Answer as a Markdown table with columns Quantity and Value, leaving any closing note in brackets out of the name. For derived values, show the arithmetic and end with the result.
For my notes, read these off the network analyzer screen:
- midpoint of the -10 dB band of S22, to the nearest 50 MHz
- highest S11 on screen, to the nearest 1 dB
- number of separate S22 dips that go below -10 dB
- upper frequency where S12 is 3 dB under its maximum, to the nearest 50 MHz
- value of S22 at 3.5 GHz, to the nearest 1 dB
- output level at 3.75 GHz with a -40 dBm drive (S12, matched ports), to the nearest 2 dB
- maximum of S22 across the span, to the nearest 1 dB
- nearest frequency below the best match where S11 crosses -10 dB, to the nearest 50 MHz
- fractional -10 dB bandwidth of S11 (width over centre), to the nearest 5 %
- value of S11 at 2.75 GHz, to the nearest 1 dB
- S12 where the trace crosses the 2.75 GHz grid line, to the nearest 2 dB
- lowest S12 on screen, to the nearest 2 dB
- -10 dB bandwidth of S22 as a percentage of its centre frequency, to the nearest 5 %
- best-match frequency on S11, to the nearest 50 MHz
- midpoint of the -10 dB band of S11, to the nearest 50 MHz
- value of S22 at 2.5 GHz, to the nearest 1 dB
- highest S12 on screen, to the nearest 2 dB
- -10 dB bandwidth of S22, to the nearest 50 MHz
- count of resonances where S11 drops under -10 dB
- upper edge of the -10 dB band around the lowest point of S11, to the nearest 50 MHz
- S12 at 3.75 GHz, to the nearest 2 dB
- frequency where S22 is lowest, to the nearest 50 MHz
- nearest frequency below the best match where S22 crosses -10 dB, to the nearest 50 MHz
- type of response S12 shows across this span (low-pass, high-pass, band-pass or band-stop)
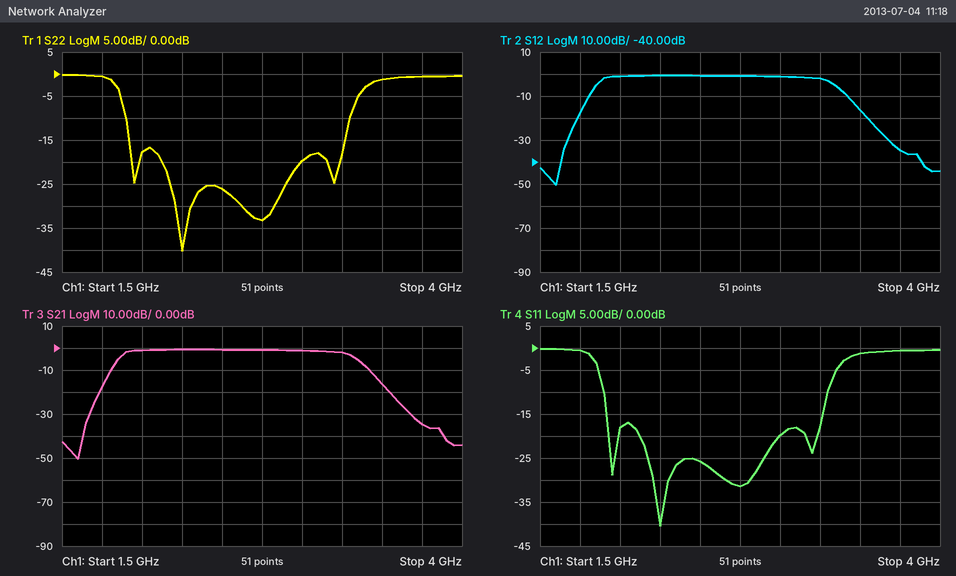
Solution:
| Quantity | Value |
|---|---|
| midpoint of the -10 dB band of S22, to the nearest 50 MHz | 2.60 GHz |
| highest S11 on screen, to the nearest 1 dB | 0 dB |
| number of separate S22 dips that go below -10 dB | 4 |
| upper frequency where S12 is 3 dB under its maximum, to the nearest 50 MHz | 3.30 GHz |
| value of S22 at 3.5 GHz, to the nearest 1 dB | -1 dB |
| output level at 3.75 GHz with a -40 dBm drive (S12, matched ports), to the nearest 2 dB | -40 dBm + (-34 dB) = -74 dBm |
| maximum of S22 across the span, to the nearest 1 dB | 0 dB |
| nearest frequency below the best match where S11 crosses -10 dB, to the nearest 50 MHz | 1.90 GHz |
| fractional -10 dB bandwidth of S11 (width over centre), to the nearest 5 % | 1.4 GHz / 2.6 GHz ≈ 53.8 %, so 55 % to the nearest 5 % |
| value of S11 at 2.75 GHz, to the nearest 1 dB | -31 dB |
| S12 where the trace crosses the 2.75 GHz grid line, to the nearest 2 dB | 0 dB |
| lowest S12 on screen, to the nearest 2 dB | -50 dB |
| -10 dB bandwidth of S22 as a percentage of its centre frequency, to the nearest 5 % | 1.4 GHz / 2.6 GHz ≈ 53.8 %, so 55 % to the nearest 5 % |
| best-match frequency on S11, to the nearest 50 MHz | 2.25 GHz |
| midpoint of the -10 dB band of S11, to the nearest 50 MHz | 2.60 GHz |
| value of S22 at 2.5 GHz, to the nearest 1 dB | -26 dB |
| highest S12 on screen, to the nearest 2 dB | 0 dB |
| -10 dB bandwidth of S22, to the nearest 50 MHz | 3.30 GHz − 1.90 GHz = 1.40 GHz |
| count of resonances where S11 drops under -10 dB | 4 |
| upper edge of the -10 dB band around the lowest point of S11, to the nearest 50 MHz | 3.30 GHz |
| S12 at 3.75 GHz, to the nearest 2 dB | -34 dB |
| frequency where S22 is lowest, to the nearest 50 MHz | 2.25 GHz |
| nearest frequency below the best match where S22 crosses -10 dB, to the nearest 50 MHz | 1.90 GHz |
| type of response S12 shows across this span | band-pass |
